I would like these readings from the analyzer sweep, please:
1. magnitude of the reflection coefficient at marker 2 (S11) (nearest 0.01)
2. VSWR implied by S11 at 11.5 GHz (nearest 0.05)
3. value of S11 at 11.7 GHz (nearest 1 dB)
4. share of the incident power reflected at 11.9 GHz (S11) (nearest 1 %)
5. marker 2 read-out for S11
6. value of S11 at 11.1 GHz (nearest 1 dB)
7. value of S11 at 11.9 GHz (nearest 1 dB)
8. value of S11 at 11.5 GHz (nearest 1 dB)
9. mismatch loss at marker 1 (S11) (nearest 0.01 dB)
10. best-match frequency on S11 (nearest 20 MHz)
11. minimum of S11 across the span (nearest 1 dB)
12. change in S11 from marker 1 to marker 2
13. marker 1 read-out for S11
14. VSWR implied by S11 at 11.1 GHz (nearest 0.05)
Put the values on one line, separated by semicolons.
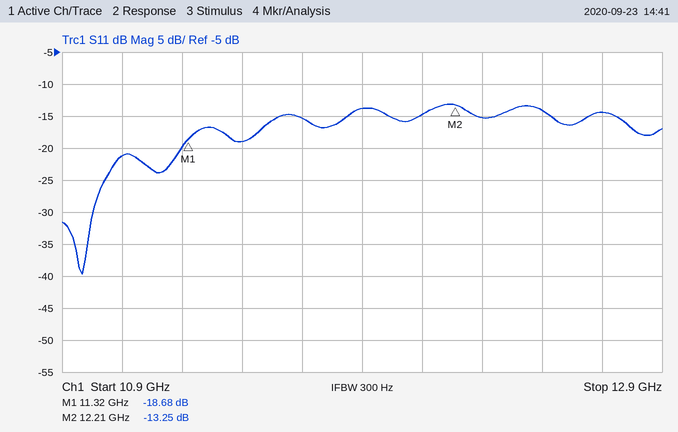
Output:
0.22; 1.25; -15 dB; 4 %; -13.25 dB; -21 dB; -14 dB; -19 dB; 0.06 dB; 10.96 GHz; -40 dB; 5.43 dB; -18.68 dB; 1.20
